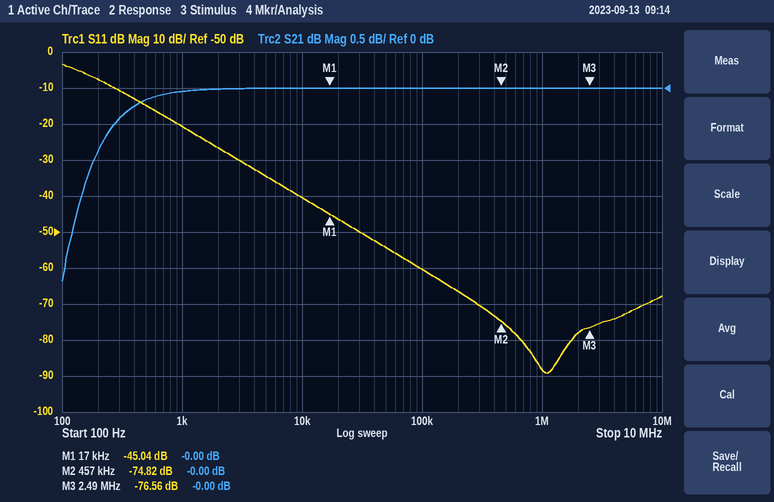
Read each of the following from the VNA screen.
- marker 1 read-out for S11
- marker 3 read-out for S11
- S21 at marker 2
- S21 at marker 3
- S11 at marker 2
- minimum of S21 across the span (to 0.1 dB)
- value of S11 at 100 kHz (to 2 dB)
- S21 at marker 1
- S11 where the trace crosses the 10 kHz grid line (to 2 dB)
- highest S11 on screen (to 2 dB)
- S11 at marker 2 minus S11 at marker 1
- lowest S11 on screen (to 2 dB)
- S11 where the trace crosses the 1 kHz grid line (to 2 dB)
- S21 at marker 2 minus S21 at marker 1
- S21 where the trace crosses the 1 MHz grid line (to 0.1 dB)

-45.04 dB
-76.56 dB
-0.00 dB
-0.00 dB
-74.82 dB
-2.7 dB
-60 dB
-0.00 dB
-40 dB
-4 dB
-29.78 dB
-90 dB
-20 dB
0.00 dB
0.0 dB
